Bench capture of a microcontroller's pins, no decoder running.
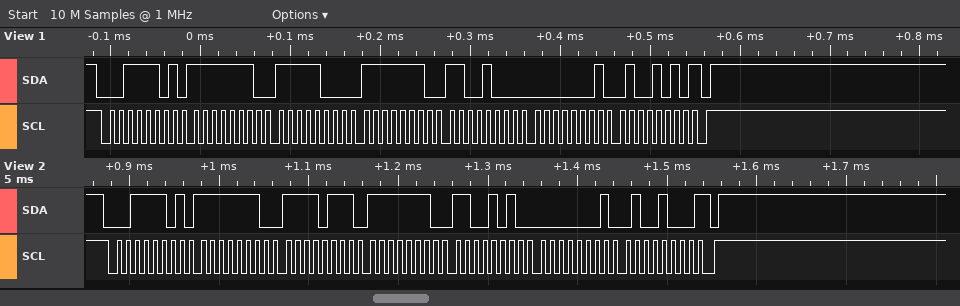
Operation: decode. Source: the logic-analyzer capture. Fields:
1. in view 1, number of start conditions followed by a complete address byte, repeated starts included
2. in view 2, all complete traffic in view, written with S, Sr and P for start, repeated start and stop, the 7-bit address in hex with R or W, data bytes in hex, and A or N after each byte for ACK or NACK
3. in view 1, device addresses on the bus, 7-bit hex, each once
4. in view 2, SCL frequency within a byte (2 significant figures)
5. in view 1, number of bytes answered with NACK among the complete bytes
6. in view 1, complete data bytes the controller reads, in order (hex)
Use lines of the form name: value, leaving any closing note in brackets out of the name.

in view 1, number of start conditions followed by a complete address byte, repeated starts included: 1
in view 2, all complete traffic in view, written with S, Sr and P for start, repeated start and stop, the 7-bit address in hex with R or W, data bytes in hex, and A or N after each byte for ACK or NACK: S 1ER A FE A F7 A FE A CA A 01 A 48 N P
in view 1, device addresses on the bus, 7-bit hex, each once: 0x1E
in view 2, SCL frequency within a byte: 100 kHz
in view 1, number of bytes answered with NACK among the complete bytes: 1
in view 1, complete data bytes the controller reads, in order: FE F8 FE C8 01 4A
